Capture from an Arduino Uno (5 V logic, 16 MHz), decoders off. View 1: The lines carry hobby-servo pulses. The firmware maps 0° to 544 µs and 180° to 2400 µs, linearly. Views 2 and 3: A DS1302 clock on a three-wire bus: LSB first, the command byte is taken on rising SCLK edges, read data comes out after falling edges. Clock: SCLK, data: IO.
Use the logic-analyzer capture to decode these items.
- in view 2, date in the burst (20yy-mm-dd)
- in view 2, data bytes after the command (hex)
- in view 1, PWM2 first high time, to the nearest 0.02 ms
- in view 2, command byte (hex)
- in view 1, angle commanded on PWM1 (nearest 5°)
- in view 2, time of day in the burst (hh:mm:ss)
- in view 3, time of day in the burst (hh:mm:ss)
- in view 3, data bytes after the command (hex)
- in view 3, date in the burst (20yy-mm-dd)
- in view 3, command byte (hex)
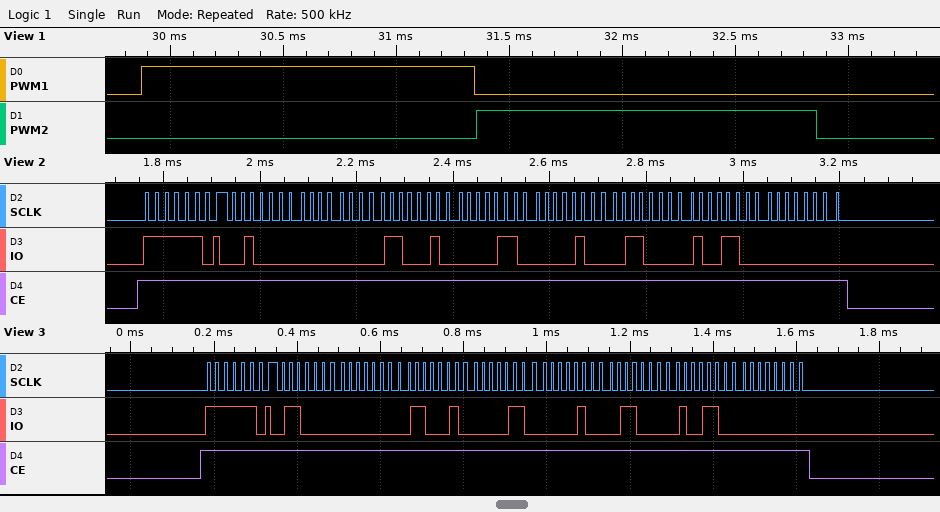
2019-10-30
04 00 23 30 10 06 19 00
1.50 ms
0xBF
90°
23:00:04
23:00:06
06 00 23 30 10 06 19 00
2019-10-30
0xBF
